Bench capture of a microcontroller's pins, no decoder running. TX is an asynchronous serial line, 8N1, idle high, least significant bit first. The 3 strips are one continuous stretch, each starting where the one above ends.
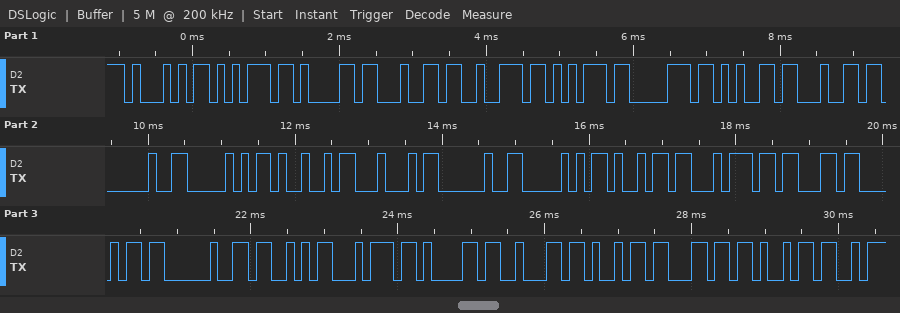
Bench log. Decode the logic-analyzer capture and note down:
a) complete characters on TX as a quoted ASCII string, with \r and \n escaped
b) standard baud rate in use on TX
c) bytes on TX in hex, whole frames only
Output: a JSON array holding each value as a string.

["\"Quadruped PID Pitch Stabili\"", "9600 baud", "51 75 61 64 72 75 70 65 64 20 50 49 44 20 50 69 74 63 68 20 53 74 61 62 69 6C 69"]
